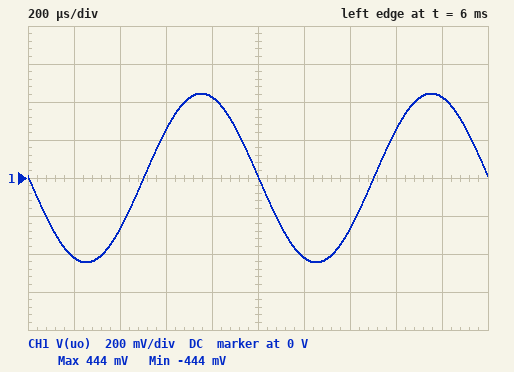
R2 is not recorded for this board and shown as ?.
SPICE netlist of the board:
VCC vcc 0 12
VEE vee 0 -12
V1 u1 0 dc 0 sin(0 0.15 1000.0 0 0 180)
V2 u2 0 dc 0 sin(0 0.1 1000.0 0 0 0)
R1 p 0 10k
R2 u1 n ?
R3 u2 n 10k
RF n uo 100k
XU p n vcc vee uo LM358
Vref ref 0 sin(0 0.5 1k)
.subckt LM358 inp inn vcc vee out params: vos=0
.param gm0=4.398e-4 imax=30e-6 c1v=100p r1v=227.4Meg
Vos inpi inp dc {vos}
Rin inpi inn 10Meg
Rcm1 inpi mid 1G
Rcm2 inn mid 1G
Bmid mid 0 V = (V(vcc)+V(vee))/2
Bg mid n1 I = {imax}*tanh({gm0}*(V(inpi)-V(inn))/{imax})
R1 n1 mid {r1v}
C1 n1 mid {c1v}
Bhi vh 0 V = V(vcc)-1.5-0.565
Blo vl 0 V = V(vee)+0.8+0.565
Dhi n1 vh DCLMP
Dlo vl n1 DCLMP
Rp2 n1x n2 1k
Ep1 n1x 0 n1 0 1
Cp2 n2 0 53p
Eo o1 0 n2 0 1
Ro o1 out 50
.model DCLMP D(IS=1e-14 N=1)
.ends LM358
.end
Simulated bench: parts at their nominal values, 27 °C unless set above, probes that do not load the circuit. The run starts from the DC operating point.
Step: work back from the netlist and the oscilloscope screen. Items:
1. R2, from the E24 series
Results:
27 kΩ
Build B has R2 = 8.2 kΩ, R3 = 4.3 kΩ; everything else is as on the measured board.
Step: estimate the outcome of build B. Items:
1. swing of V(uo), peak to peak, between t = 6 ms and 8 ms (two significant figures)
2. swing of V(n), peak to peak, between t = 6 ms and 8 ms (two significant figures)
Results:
990 mV
1.4 mV
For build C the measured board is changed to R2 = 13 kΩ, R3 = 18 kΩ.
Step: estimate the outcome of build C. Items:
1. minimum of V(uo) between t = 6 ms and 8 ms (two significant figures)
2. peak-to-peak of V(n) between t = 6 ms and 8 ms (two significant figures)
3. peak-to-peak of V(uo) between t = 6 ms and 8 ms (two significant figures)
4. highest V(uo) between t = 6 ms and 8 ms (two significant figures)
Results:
-600 mV
1.7 mV
1.2 V
600 mV
